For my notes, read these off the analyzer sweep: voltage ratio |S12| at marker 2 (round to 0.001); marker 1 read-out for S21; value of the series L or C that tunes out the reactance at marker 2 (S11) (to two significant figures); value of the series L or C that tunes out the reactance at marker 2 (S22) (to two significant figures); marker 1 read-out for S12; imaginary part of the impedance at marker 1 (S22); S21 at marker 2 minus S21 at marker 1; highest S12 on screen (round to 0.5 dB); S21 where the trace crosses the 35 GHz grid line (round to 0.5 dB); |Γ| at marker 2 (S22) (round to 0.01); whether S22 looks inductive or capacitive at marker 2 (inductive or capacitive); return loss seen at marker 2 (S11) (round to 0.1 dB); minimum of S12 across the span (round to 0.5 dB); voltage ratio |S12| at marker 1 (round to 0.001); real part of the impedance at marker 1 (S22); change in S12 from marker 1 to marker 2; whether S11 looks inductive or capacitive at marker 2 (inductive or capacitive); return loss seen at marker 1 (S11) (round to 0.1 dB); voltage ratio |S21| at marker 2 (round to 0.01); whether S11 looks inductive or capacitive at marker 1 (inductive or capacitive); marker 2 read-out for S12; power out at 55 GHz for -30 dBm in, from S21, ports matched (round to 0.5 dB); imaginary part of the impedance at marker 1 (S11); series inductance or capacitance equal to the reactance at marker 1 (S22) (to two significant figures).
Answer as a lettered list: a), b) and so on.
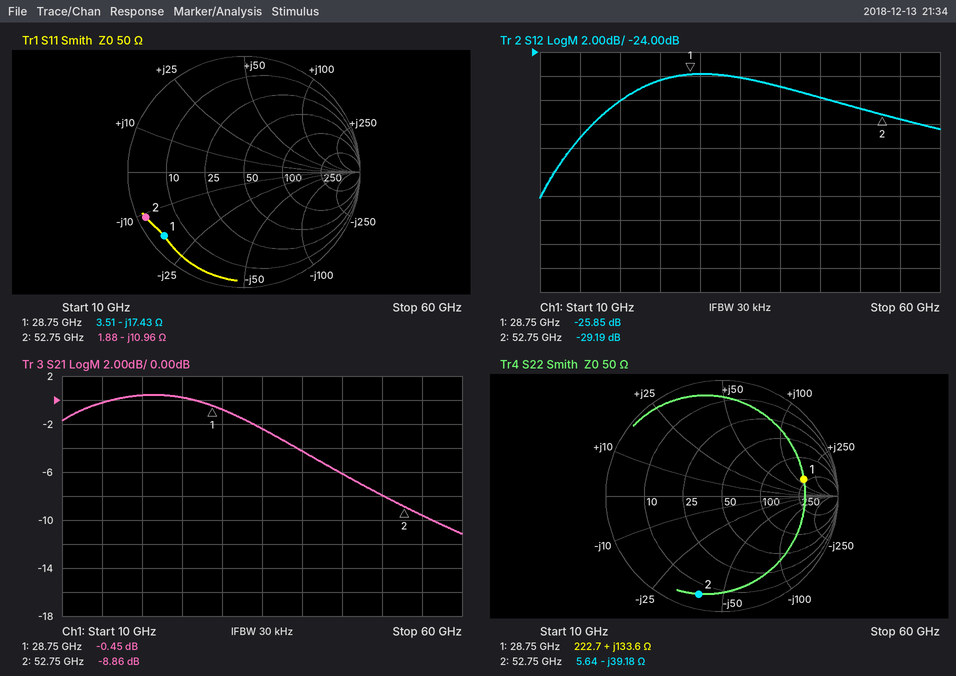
a) 0.035
b) -0.45 dB
c) 33 pH
d) 120 pH
e) -25.85 dB
f) +133.6 Ω
g) -8.41 dB
h) -26.0 dB
i) -2.5 dB
j) 0.87
k) capacitive
l) 0.6 dB
m) -36.0 dB
n) 0.051
o) 222.7 Ω
p) -3.34 dB
q) capacitive
r) 1.1 dB
s) 0.36
t) capacitive
u) -29.19 dB
v) -39.5 dBm
w) -17.43 Ω
x) 740 pH
